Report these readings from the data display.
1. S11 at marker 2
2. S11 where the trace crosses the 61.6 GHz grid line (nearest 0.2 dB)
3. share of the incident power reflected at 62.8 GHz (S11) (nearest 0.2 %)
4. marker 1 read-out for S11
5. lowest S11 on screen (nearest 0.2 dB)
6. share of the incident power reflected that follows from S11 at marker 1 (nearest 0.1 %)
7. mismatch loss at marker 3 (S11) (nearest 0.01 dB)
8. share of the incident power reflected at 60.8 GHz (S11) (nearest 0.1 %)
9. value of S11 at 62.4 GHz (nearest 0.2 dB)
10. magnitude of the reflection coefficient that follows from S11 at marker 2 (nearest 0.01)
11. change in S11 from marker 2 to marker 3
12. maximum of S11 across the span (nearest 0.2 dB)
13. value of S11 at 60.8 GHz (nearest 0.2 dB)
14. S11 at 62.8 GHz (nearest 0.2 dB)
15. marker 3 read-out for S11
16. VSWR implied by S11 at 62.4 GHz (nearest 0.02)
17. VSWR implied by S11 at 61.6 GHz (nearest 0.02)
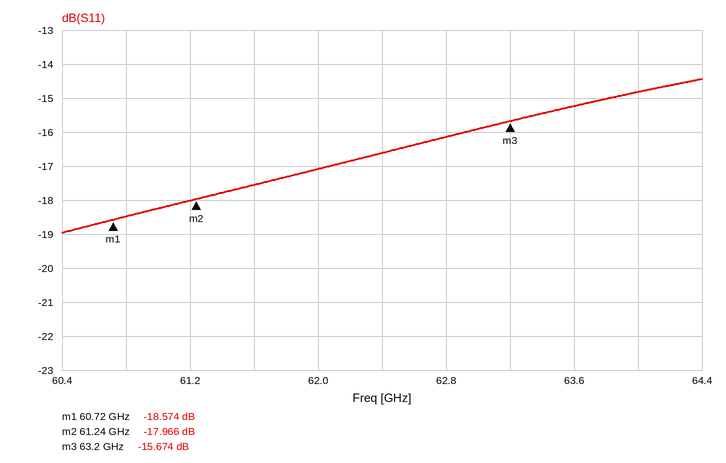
-17.966 dB
-17.6 dB
2.4 %
-18.574 dB
-19.0 dB
1.4 %
0.12 dB
1.4 %
-16.6 dB
0.13
2.292 dB
-14.4 dB
-18.4 dB
-16.2 dB
-15.674 dB
1.34
1.30
